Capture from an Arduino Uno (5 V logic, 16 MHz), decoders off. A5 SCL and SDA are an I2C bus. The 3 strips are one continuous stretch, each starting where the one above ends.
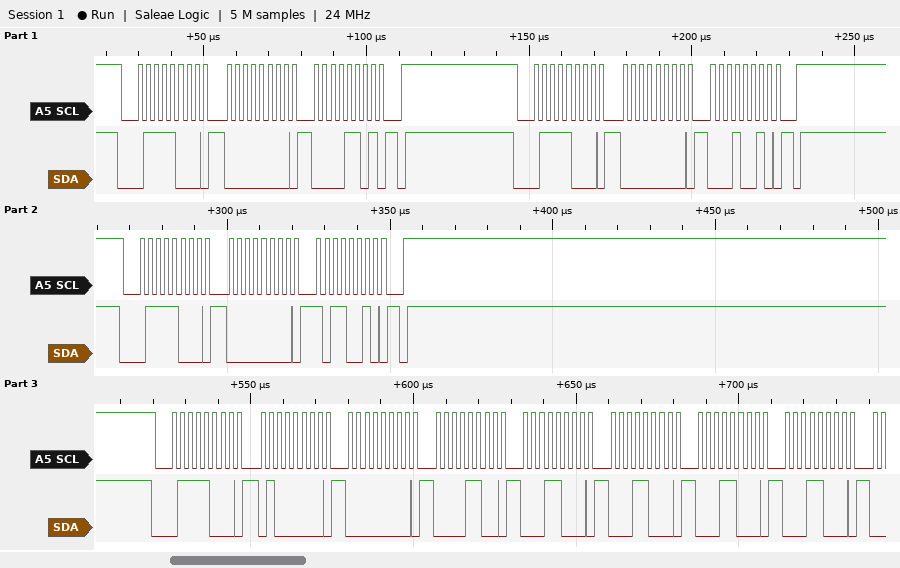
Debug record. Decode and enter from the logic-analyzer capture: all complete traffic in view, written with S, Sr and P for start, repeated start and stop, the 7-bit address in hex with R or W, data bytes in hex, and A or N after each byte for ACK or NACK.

S 3CW A 00 A 0D A P S 3CW A 00 A 12 A P S 3CW A 00 A B2 A P S 3CW A 40 A 00 A 0C A 18 A 18 A 18 A 18 A
